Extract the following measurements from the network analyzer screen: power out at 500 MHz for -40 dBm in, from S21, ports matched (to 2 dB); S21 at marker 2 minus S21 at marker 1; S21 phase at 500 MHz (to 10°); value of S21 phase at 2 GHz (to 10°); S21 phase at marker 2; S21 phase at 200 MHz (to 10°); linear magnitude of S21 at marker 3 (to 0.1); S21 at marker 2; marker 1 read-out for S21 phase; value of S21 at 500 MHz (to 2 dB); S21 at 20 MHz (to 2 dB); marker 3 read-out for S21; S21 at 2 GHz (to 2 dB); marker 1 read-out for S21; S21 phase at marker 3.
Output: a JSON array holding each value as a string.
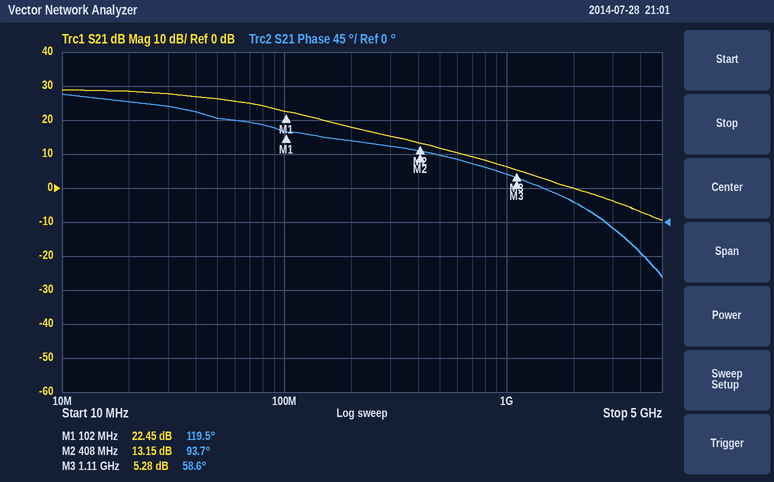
["-28 dBm", "-9.30 dB", "90°", "30°", "93.7°", "110°", "1.8", "13.15 dB", "119.5°", "12 dB", "28 dB", "5.28 dB", "0 dB", "22.45 dB", "58.6°"]
